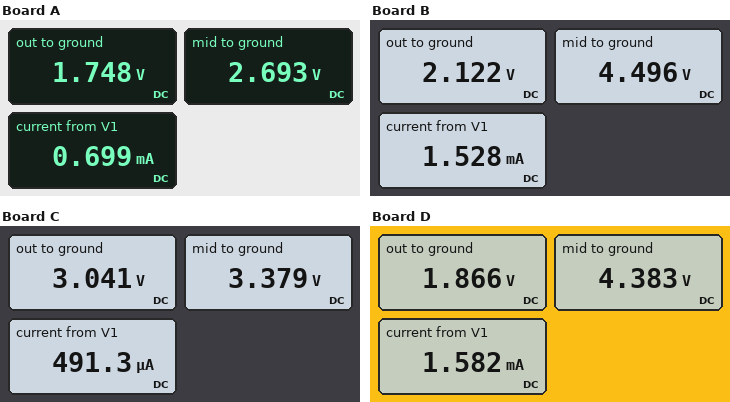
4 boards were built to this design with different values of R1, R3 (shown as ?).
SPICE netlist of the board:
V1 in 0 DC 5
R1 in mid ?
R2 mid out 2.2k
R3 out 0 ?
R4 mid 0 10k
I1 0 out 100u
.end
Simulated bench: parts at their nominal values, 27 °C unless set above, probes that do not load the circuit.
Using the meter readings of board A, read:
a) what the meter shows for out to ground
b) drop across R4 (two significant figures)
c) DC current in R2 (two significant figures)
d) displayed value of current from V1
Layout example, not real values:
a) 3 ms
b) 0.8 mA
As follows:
a) 1.748 V
b) 2.7 V
c) 430 µA
d) 0.699 mA
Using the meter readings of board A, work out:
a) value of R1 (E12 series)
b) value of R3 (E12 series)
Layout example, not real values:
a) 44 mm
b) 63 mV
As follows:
a) 3.3 kΩ
b) 3.3 kΩ
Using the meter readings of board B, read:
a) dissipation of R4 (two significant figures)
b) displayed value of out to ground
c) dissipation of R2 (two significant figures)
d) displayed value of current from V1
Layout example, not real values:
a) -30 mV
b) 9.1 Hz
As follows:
a) 2.0 mW
b) 2.122 V
c) 2.6 mW
d) 1.528 mA
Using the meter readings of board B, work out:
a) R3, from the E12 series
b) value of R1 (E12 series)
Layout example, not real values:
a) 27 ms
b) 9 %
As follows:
a) 1.8 kΩ
b) 330 Ω
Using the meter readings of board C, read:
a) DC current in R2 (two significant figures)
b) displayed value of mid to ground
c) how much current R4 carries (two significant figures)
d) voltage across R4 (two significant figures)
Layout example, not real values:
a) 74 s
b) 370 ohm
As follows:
a) 150 µA
b) 3.379 V
c) 340 µA
d) 3.4 V
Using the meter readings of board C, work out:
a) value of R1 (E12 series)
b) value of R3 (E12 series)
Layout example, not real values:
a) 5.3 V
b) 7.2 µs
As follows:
a) 3.3 kΩ
b) 12 kΩ
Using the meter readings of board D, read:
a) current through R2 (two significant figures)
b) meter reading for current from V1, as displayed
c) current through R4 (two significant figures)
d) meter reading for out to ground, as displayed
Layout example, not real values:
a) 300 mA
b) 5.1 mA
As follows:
a) 1.1 mA
b) 1.582 mA
c) 440 µA
d) 1.866 V
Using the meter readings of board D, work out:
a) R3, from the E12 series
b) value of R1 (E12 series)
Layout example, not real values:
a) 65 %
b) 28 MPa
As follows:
a) 1.5 kΩ
b) 390 Ω
